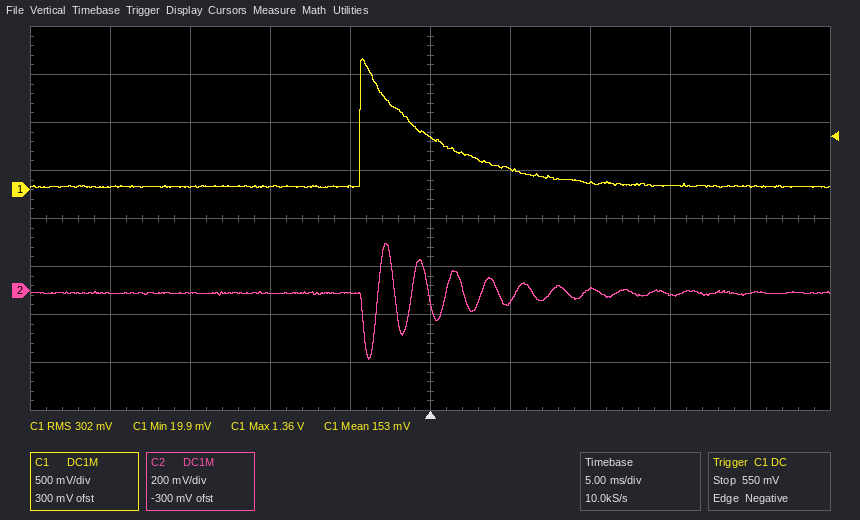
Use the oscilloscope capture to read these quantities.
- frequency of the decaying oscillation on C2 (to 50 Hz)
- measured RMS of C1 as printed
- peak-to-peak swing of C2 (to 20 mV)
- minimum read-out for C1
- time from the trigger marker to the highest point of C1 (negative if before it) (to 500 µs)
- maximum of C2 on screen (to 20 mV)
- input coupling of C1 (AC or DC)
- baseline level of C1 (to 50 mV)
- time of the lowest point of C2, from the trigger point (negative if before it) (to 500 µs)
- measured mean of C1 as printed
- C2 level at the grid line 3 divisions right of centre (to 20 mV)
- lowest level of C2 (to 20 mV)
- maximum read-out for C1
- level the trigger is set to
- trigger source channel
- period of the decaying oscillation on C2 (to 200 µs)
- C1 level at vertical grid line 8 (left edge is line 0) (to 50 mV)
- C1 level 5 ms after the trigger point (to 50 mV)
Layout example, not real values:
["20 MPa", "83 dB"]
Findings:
["450 Hz", "302 mV", "480 mV", "19.9 mV", "-4.0 ms", "200 mV", "DC", "50 mV", "-4.0 ms", "153 mV", "-20 mV", "-280 mV", "1.36 V", "550 mV", "C1", "2.2 ms", "50 mV", "200 mV"]
